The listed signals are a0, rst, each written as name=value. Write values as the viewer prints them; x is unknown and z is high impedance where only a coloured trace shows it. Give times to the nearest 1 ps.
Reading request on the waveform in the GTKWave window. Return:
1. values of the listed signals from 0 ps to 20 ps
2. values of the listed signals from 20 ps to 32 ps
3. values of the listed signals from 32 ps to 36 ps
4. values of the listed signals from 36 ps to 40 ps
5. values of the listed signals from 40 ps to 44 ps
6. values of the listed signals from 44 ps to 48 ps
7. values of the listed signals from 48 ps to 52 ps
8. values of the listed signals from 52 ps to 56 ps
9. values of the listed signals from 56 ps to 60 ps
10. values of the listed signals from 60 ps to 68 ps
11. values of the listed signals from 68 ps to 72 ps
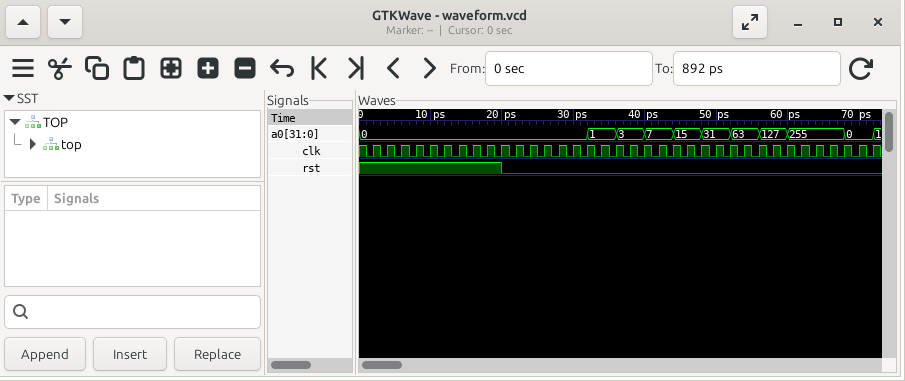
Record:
a0=0, rst=1
a0=0, rst=0
a0=1, rst=0
a0=3, rst=0
a0=7, rst=0
a0=15, rst=0
a0=31, rst=0
a0=63, rst=0
a0=127, rst=0
a0=255, rst=0
a0=0, rst=0
